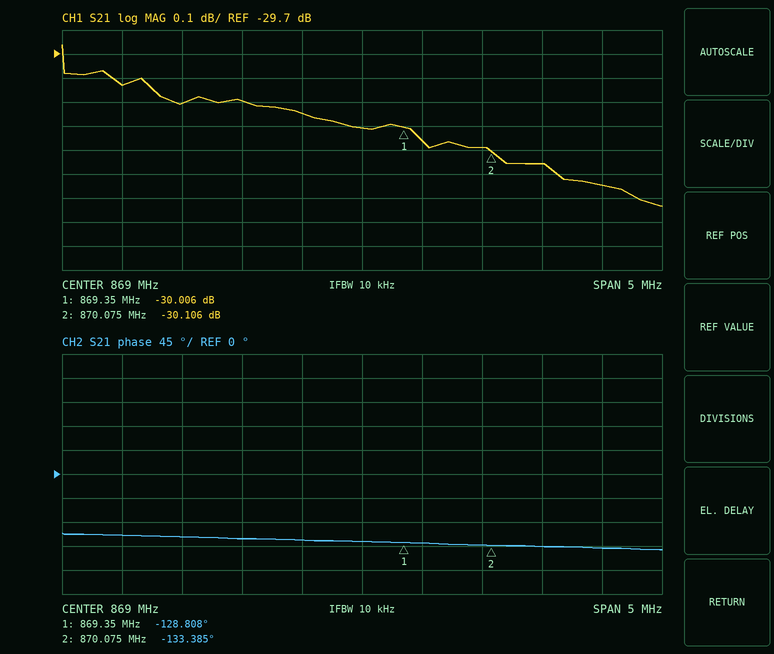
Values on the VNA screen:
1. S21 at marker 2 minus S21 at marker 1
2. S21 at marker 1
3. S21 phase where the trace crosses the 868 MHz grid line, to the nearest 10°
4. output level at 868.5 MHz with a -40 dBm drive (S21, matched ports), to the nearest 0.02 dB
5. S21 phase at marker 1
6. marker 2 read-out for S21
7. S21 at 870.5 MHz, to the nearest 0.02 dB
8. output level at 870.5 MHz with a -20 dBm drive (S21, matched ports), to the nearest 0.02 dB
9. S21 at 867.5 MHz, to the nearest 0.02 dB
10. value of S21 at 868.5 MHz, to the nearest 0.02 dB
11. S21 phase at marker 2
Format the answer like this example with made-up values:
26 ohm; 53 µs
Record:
-0.100 dB; -30.006 dB; -120°; -69.94 dBm; -128.808°; -30.106 dB; -30.16 dB; -50.16 dBm; -29.90 dB; -29.94 dB; -133.385°
